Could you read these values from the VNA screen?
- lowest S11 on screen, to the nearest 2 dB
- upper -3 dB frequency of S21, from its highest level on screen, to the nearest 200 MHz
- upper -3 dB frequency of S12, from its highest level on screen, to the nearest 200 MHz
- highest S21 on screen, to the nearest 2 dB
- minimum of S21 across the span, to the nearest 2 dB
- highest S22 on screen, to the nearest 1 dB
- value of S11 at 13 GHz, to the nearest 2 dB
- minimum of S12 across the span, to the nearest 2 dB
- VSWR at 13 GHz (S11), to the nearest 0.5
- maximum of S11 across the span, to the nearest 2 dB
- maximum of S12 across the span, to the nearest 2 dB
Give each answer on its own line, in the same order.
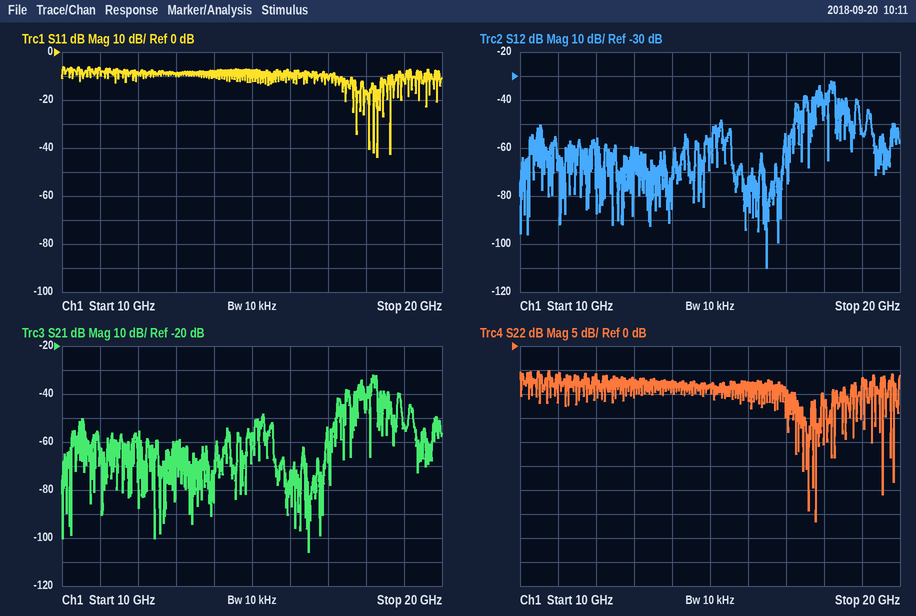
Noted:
-44 dB
18.2 GHz
18.2 GHz
-32 dB
-106 dB
-5 dB
-10 dB
-110 dB
2.0
-6 dB
-32 dB
